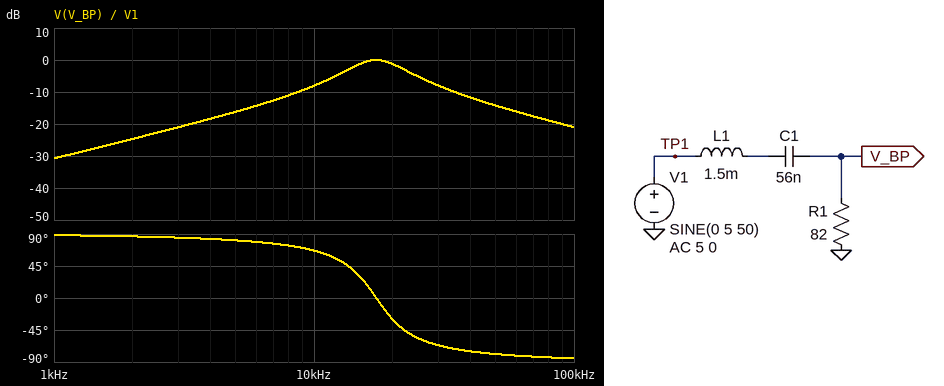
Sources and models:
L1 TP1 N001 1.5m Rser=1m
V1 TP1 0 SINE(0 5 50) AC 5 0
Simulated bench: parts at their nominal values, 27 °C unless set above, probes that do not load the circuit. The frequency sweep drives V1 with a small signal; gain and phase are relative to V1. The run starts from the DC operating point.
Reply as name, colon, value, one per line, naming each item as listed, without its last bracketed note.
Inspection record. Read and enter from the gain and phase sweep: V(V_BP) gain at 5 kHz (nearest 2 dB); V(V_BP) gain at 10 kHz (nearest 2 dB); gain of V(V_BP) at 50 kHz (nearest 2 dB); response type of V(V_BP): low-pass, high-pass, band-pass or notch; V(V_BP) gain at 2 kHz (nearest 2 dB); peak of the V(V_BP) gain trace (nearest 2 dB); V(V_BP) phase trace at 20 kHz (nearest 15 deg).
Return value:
V(V_BP) gain at 5 kHz: -16 dB
V(V_BP) gain at 10 kHz: -8 dB
gain of V(V_BP) at 50 kHz: -14 dB
response type of V(V_BP): low-pass, high-pass, band-pass or notch: band-pass
V(V_BP) gain at 2 kHz: -24 dB
peak of the V(V_BP) gain trace: 0 dB
V(V_BP) phase trace at 20 kHz: -30 deg
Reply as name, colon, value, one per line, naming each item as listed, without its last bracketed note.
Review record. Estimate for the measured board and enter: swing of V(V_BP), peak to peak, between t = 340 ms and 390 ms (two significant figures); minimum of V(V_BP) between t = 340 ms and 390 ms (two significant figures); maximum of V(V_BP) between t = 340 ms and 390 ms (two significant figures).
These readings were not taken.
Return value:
swing of V(V_BP), peak to peak, between t = 340 ms and 390 ms: 14 mV
minimum of V(V_BP) between t = 340 ms and 390 ms: -7.2 mV
maximum of V(V_BP) between t = 340 ms and 390 ms: 7.2 mV
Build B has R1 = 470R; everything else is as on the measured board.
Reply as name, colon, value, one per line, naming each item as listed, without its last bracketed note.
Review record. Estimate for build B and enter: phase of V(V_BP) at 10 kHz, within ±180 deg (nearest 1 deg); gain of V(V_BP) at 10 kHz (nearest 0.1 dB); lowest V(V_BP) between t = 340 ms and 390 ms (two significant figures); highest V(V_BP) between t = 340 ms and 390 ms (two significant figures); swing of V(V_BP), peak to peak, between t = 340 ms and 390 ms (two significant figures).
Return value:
phase of V(V_BP) at 10 kHz, within ±180 deg: 22 deg
gain of V(V_BP) at 10 kHz: -0.7 dB
lowest V(V_BP) between t = 340 ms and 390 ms: -41 mV
highest V(V_BP) between t = 340 ms and 390 ms: 41 mV
swing of V(V_BP), peak to peak, between t = 340 ms and 390 ms: 83 mV
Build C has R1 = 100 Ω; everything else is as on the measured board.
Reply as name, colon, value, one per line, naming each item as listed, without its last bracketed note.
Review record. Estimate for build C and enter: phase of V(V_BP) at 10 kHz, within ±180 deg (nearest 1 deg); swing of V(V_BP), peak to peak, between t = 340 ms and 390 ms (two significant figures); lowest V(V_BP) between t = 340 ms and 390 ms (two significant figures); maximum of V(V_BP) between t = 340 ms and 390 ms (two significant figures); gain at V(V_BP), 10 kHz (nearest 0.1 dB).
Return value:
phase of V(V_BP) at 10 kHz, within ±180 deg: 62 deg
swing of V(V_BP), peak to peak, between t = 340 ms and 390 ms: 18 mV
lowest V(V_BP) between t = 340 ms and 390 ms: -8.8 mV
maximum of V(V_BP) between t = 340 ms and 390 ms: 8.8 mV
gain at V(V_BP), 10 kHz: -6.6 dB
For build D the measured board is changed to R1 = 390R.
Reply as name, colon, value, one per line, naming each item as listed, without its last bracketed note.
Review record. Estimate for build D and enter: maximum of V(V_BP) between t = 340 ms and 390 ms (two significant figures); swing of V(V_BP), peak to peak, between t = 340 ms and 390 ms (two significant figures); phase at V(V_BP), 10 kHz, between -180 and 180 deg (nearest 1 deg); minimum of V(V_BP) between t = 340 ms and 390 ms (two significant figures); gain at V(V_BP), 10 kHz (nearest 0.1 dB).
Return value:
maximum of V(V_BP) between t = 340 ms and 390 ms: 34 mV
swing of V(V_BP), peak to peak, between t = 340 ms and 390 ms: 69 mV
phase at V(V_BP), 10 kHz, between -180 and 180 deg: 26 deg
minimum of V(V_BP) between t = 340 ms and 390 ms: -34 mV
gain at V(V_BP), 10 kHz: -0.9 dB
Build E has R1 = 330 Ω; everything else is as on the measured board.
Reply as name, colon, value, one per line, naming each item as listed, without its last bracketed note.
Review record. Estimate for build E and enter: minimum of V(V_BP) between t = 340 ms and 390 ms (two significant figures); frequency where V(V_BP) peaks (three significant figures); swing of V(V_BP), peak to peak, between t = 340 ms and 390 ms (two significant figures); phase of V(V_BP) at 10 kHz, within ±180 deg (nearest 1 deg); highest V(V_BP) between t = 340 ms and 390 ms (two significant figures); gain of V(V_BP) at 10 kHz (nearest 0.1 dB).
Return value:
minimum of V(V_BP) between t = 340 ms and 390 ms: -29 mV
frequency where V(V_BP) peaks: 17.4 kHz
swing of V(V_BP), peak to peak, between t = 340 ms and 390 ms: 58 mV
phase of V(V_BP) at 10 kHz, within ±180 deg: 30 deg
highest V(V_BP) between t = 340 ms and 390 ms: 29 mV
gain of V(V_BP) at 10 kHz: -1.2 dB
